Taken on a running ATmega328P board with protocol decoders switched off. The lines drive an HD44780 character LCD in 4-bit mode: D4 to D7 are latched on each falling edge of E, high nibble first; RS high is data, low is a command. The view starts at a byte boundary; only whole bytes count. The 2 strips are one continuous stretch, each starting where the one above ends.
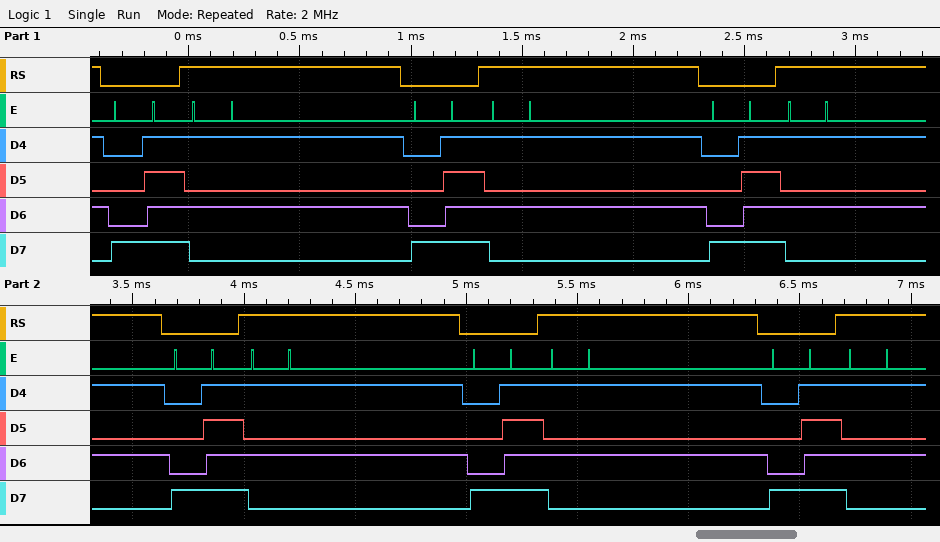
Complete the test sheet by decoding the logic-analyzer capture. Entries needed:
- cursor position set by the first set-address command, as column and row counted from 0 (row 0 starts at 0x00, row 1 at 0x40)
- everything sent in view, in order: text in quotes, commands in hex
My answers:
column 15, row 0
0x8F "U" 0x8F "U" 0x8F "U" 0x8F "U" 0x8F "U" 0x8F "U"
